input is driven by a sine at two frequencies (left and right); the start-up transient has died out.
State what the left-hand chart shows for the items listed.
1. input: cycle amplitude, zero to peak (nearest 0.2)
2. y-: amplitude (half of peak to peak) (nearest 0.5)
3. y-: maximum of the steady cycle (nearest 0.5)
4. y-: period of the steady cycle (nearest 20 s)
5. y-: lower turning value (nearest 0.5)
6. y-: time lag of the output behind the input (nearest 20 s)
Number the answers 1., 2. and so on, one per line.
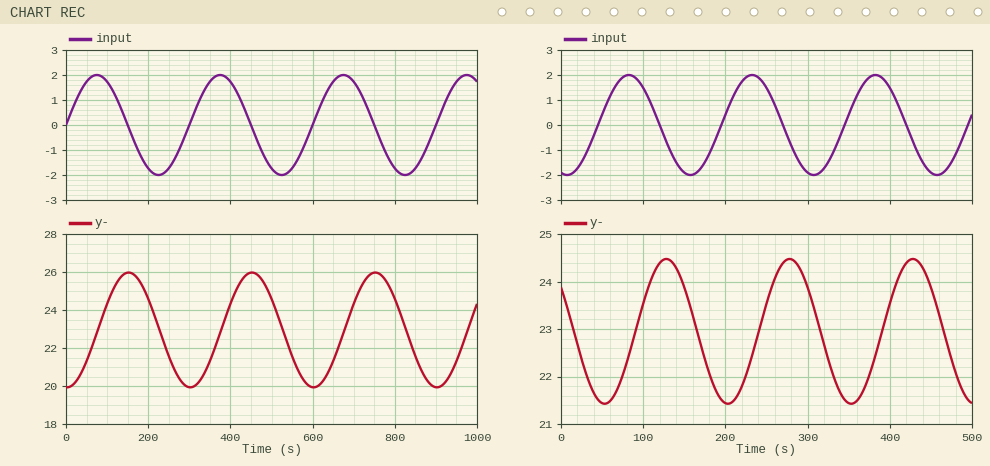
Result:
1. 2.0
2. 3.0
3. 26.0
4. 300 s
5. 20.0
6. 80 s
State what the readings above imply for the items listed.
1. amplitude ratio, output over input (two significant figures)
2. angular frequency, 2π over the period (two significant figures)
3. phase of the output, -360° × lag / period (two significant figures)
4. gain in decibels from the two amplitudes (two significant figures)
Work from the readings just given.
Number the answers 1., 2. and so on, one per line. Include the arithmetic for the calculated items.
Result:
1. 3 / 2 = 1.5
2. 2π / 300 = 0.021 rad/s
3. -360 × 80 / 300 = -96°
4. 20 log10(3 / 2) = 3.5 dB
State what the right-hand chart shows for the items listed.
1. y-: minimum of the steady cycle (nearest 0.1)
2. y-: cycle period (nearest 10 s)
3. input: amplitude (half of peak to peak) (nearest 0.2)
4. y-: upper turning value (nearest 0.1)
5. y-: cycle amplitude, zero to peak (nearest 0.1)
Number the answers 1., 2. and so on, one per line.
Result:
1. 21.4
2. 150 s
3. 2.0
4. 24.5
5. 1.5
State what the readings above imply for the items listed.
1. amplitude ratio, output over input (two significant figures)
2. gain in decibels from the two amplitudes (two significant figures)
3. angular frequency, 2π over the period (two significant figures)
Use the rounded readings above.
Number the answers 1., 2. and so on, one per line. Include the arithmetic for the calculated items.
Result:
1. 1.5 / 2 = 0.75
2. 20 log10(1.5 / 2) = -2.5 dB
3. 2π / 150 = 0.042 rad/s
